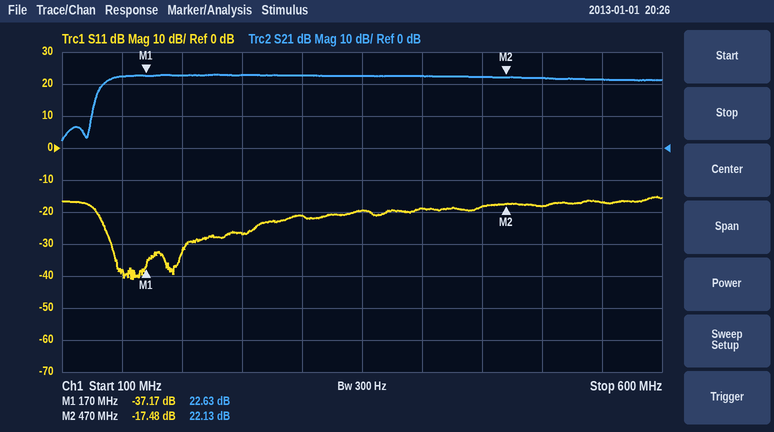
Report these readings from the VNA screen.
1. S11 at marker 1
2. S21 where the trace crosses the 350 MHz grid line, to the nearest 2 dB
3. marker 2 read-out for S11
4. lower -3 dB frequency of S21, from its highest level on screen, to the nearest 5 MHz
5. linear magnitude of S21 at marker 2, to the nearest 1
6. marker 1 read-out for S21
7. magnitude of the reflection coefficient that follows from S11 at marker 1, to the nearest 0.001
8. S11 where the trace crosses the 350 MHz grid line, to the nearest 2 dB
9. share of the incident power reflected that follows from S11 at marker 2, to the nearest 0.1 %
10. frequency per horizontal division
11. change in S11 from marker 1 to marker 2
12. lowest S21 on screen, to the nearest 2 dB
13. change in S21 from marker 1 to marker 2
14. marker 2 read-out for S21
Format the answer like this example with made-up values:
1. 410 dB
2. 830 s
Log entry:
1. -37.17 dB
2. 22 dB
3. -17.48 dB
4. 135 MHz
5. 13
6. 22.63 dB
7. 0.014
8. -20 dB
9. 1.8 %
10. 50 MHz
11. 19.69 dB
12. 2 dB
13. -0.50 dB
14. 22.13 dB
